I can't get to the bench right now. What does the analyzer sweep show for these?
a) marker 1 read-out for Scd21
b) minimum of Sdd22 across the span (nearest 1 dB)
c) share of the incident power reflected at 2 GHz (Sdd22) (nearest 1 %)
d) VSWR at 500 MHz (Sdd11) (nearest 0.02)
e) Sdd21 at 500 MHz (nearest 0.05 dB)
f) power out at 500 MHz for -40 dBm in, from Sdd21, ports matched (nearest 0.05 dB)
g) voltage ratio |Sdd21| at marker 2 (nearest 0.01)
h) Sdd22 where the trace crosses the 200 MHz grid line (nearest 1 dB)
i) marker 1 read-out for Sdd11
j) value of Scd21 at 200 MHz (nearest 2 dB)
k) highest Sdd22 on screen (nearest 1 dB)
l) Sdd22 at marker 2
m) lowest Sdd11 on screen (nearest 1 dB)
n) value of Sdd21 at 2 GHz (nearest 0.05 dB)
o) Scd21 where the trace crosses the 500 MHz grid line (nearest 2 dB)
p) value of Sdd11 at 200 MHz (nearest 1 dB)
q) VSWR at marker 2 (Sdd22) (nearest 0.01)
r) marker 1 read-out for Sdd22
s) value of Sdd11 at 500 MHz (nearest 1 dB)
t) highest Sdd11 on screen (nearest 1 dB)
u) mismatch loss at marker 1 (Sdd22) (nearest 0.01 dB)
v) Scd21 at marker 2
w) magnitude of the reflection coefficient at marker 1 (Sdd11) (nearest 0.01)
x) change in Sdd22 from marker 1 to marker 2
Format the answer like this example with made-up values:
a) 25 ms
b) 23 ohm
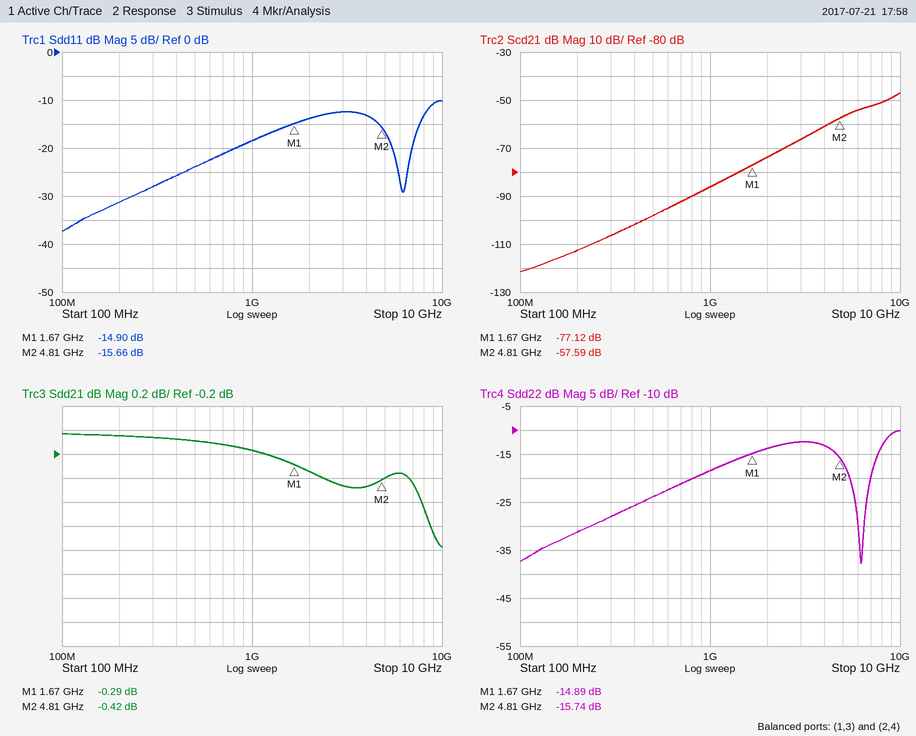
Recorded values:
a) -77.12 dB
b) -38 dB
c) 4 %
d) 1.14
e) -0.10 dB
f) -40.10 dBm
g) 0.95
h) -31 dB
i) -14.90 dB
j) -112 dB
k) -10 dB
l) -15.74 dB
m) -37 dB
n) -0.35 dB
o) -98 dB
p) -31 dB
q) 1.39
r) -14.89 dB
s) -24 dB
t) -10 dB
u) 0.14 dB
v) -57.59 dB
w) 0.18
x) -0.85 dB
